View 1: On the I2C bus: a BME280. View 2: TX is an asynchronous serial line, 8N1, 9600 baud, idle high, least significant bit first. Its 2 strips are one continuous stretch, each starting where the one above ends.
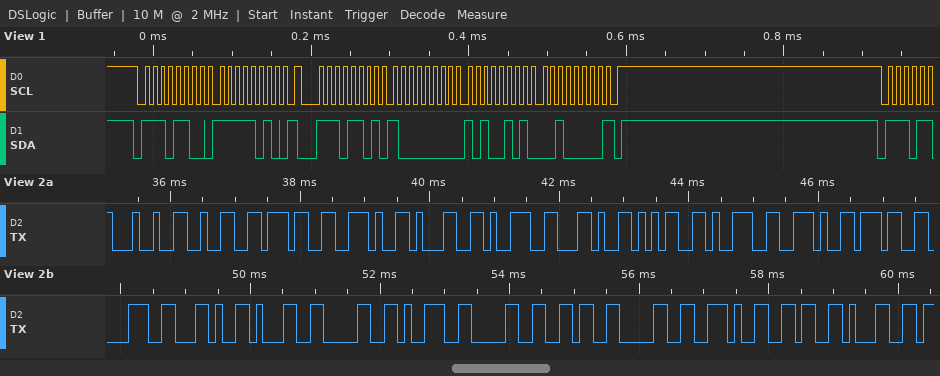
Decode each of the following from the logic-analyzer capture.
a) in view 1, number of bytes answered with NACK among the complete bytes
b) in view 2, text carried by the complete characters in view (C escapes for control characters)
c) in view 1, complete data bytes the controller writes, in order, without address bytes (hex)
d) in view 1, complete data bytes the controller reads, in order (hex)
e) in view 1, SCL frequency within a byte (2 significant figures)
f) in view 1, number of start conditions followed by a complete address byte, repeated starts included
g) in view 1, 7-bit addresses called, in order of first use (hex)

1
"$27.19,59.78,109060.61"
FA
80 A5 20
100 kHz
2
0x76
